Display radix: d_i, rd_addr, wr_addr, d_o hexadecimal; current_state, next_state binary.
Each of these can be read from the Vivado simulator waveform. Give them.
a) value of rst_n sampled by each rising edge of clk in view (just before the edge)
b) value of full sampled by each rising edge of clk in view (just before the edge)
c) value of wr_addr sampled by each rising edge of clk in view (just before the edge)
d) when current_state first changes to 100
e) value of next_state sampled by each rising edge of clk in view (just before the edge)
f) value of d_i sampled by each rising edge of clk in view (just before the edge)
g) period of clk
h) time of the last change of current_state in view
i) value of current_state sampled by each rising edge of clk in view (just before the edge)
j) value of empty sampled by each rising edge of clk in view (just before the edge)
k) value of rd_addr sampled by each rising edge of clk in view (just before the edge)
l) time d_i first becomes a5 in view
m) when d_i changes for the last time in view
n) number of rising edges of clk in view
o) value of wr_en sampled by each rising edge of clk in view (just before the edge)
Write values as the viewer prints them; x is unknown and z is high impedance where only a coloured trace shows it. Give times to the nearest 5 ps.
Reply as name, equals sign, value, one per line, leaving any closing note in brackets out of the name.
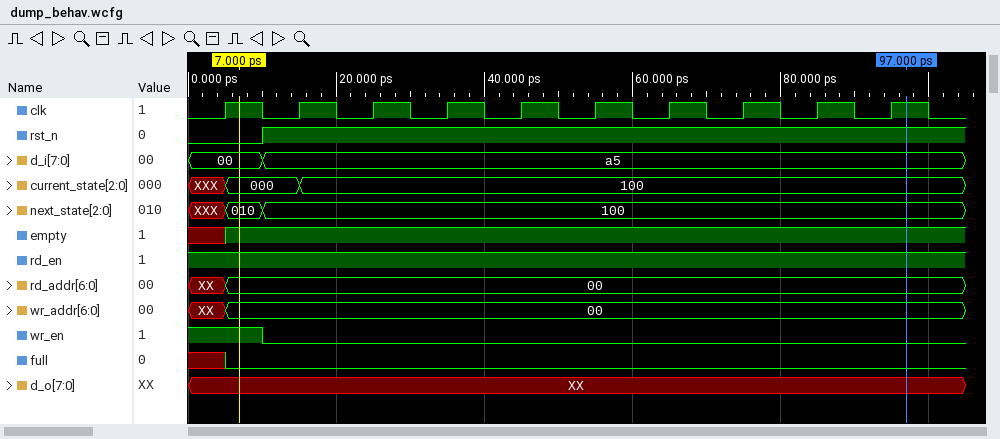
value of rst_n sampled by each rising edge of clk in view = 0 1 1 1 1 1 1 1 1 1
value of full sampled by each rising edge of clk in view = x 0 0 0 0 0 0 0 0 0
value of wr_addr sampled by each rising edge of clk in view = XX, 00, 00, 00, 00, 00, 00, 00, 00, 00
when current_state first changes to 100 = 15 ps
value of next_state sampled by each rising edge of clk in view = XXX, 100, 100, 100, 100, 100, 100, 100, 100, 100
value of d_i sampled by each rising edge of clk in view = 00, a5, a5, a5, a5, a5, a5, a5, a5, a5
period of clk = 10 ps
time of the last change of current_state in view = 15 ps
value of current_state sampled by each rising edge of clk in view = XXX, 000, 100, 100, 100, 100, 100, 100, 100, 100
value of empty sampled by each rising edge of clk in view = x 1 1 1 1 1 1 1 1 1
value of rd_addr sampled by each rising edge of clk in view = XX, 00, 00, 00, 00, 00, 00, 00, 00, 00
time d_i first becomes a5 in view = 10 ps
when d_i changes for the last time in view = 10 ps
number of rising edges of clk in view = 10
value of wr_en sampled by each rising edge of clk in view = 1 0 0 0 0 0 0 0 0 0
